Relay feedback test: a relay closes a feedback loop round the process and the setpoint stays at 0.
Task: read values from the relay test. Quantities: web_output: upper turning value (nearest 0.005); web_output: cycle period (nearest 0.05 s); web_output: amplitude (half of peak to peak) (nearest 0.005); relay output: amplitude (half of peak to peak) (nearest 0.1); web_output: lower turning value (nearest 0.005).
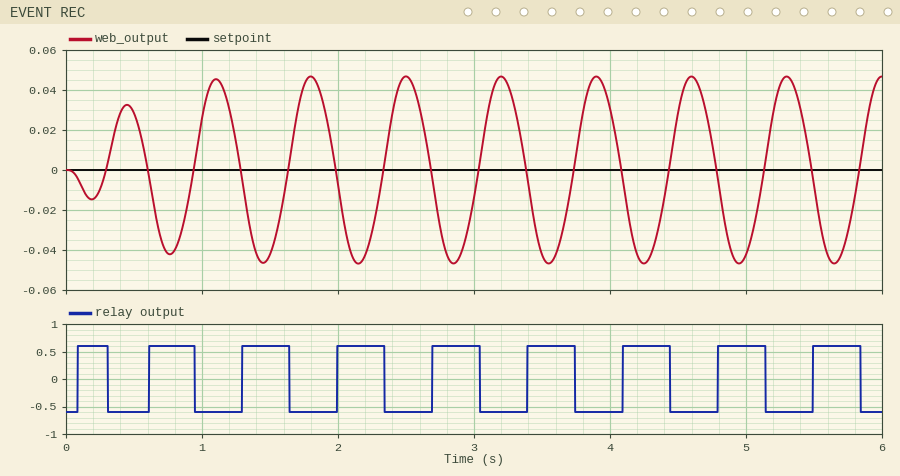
0.045
0.70 s
0.045
0.6
-0.045
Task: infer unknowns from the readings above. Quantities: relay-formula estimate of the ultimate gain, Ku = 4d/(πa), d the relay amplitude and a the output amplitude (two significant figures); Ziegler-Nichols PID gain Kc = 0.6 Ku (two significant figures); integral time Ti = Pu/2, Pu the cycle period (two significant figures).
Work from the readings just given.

17
10
0.35 s
